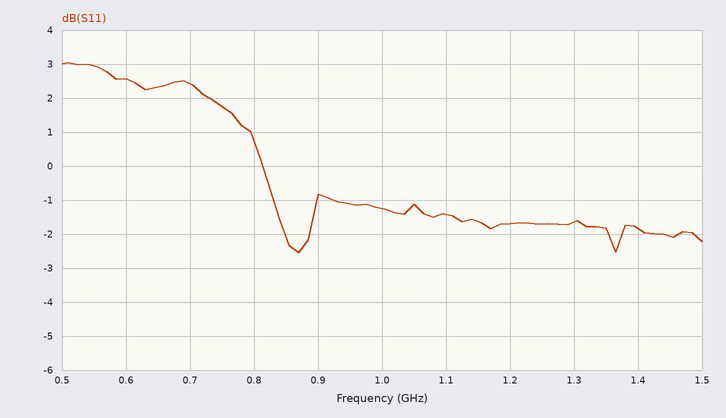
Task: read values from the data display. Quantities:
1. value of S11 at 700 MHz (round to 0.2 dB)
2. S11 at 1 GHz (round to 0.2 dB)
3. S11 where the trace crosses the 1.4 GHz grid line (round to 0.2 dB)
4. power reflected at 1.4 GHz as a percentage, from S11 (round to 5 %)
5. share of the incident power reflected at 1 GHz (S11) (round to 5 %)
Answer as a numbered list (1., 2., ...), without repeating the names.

1. 2.4 dB
2. -1.2 dB
3. -1.8 dB
4. 65 %
5. 75 %
